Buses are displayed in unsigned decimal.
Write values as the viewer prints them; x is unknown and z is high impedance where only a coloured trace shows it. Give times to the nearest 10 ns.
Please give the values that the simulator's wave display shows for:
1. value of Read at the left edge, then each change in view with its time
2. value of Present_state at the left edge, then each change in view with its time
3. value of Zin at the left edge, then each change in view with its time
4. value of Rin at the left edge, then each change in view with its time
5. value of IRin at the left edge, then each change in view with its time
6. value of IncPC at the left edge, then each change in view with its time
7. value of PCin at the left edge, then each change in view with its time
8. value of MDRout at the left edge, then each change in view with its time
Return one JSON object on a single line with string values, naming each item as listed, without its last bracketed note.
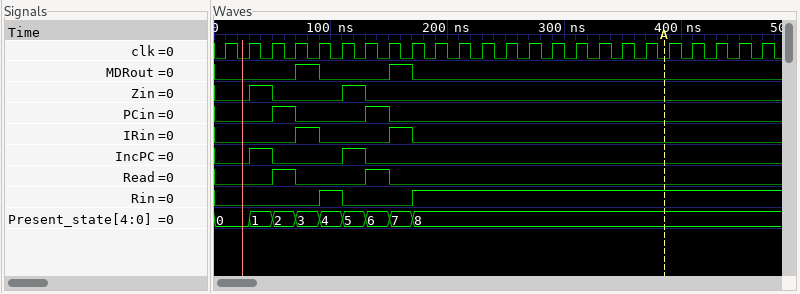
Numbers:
{"value of Read at the left edge, then each change in view with its time": "0, 1 at 50 ns, 0 at 70 ns, 1 at 130 ns, 0 at 150 ns", "value of Present_state at the left edge, then each change in view with its time": "0, 1 at 30 ns, 2 at 50 ns, 3 at 70 ns, 4 at 90 ns, 5 at 110 ns, 6 at 130 ns, 7 at 150 ns, 8 at 170 ns", "value of Zin at the left edge, then each change in view with its time": "0, 1 at 30 ns, 0 at 50 ns, 1 at 110 ns, 0 at 130 ns", "value of Rin at the left edge, then each change in view with its time": "0, 1 at 90 ns, 0 at 110 ns, 1 at 170 ns", "value of IRin at the left edge, then each change in view with its time": "0, 1 at 70 ns, 0 at 90 ns, 1 at 150 ns, 0 at 170 ns", "value of IncPC at the left edge, then each change in view with its time": "0, 1 at 30 ns, 0 at 50 ns, 1 at 110 ns, 0 at 130 ns", "value of PCin at the left edge, then each change in view with its time": "0, 1 at 50 ns, 0 at 70 ns, 1 at 130 ns, 0 at 150 ns", "value of MDRout at the left edge, then each change in view with its time": "0, 1 at 70 ns, 0 at 90 ns, 1 at 150 ns, 0 at 170 ns"}
